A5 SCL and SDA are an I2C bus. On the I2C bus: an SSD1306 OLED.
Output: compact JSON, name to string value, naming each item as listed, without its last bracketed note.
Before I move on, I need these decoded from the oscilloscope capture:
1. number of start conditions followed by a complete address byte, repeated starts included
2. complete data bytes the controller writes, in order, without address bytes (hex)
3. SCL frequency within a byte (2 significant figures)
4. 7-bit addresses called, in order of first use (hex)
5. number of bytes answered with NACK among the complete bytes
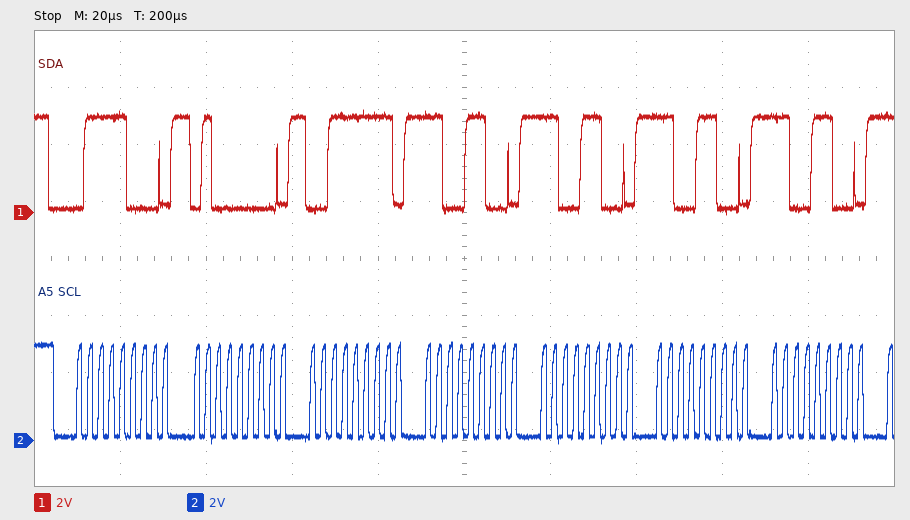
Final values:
{"number of start conditions followed by a complete address byte, repeated starts included": "1", "complete data bytes the controller writes, in order, without address bytes": "40 3F CC CC CC CC", "SCL frequency within a byte": "400 kHz", "7-bit addresses called, in order of first use": "0x3C", "number of bytes answered with NACK among the complete bytes": "0"}
